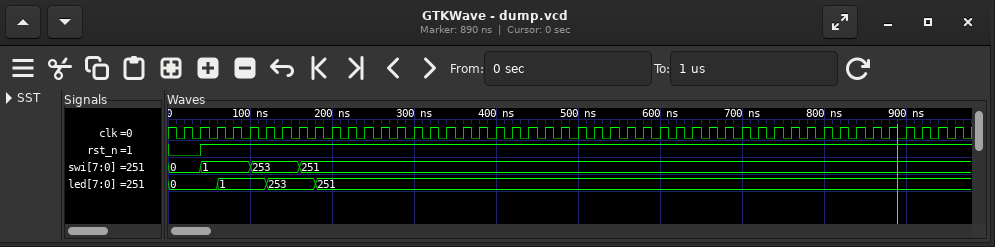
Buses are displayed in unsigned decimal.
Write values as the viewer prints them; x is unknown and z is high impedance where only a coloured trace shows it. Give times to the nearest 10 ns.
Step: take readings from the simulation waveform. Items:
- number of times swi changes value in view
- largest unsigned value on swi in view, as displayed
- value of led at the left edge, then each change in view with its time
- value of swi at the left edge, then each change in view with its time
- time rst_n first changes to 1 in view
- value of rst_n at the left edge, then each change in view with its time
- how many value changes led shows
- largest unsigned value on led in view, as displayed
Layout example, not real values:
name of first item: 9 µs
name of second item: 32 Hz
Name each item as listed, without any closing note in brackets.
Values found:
number of times swi changes value in view: 3
largest unsigned value on swi in view, as displayed: 253
value of led at the left edge, then each change in view with its time: 0, 1 at 60 ns, 253 at 120 ns, 251 at 180 ns
value of swi at the left edge, then each change in view with its time: 0, 1 at 40 ns, 253 at 100 ns, 251 at 160 ns
time rst_n first changes to 1 in view: 40 ns
value of rst_n at the left edge, then each change in view with its time: 0, 1 at 40 ns
how many value changes led shows: 3
largest unsigned value on led in view, as displayed: 253
